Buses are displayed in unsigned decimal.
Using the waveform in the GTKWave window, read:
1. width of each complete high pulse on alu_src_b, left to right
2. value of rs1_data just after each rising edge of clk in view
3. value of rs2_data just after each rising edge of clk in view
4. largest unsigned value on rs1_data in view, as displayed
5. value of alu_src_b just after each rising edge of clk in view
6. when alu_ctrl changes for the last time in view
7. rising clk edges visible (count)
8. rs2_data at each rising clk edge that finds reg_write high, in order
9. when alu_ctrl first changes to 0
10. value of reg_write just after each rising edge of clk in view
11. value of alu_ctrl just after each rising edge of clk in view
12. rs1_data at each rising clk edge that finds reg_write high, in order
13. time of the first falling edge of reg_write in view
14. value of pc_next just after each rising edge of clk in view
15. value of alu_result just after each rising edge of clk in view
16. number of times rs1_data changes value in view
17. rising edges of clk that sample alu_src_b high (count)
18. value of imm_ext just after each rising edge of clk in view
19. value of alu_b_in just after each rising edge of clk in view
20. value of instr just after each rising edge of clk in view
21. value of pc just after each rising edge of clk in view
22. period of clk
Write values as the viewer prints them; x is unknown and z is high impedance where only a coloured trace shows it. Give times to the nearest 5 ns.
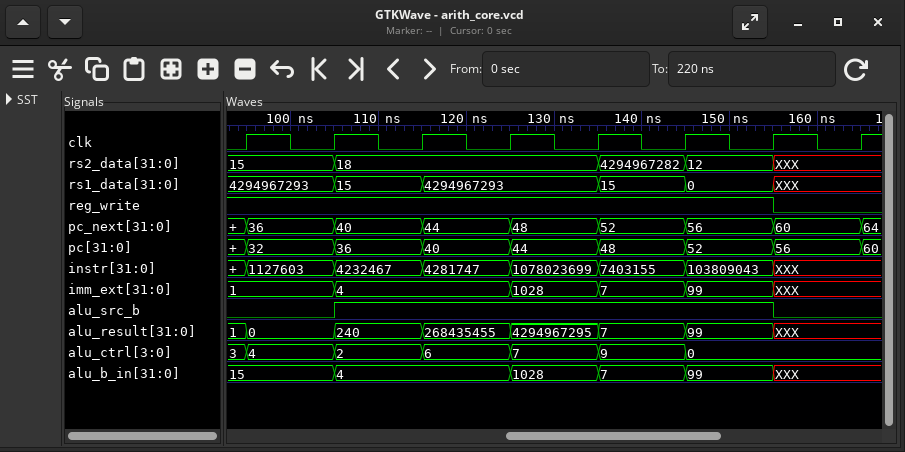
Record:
50 ns
4294967293, 15, 4294967293, 4294967293, 15, 0, XXX, XXX
15, 18, 18, 18, 4294967282, 12, XXX, XXX
4294967293
0 1 1 1 1 1 0 0
145 ns
8
15, 15, 18, 18, 18, 4294967282, 12
145 ns
1 1 1 1 1 1 0 0
4, 2, 6, 7, 9, 0, 0, 0
4294967293, 4294967293, 15, 4294967293, 4294967293, 15, 0
155 ns
36, 40, 44, 48, 52, 56, 60, 64
0, 240, 268435455, 4294967295, 7, 99, XXX, XXX
5
5
1, 4, 4, 1028, 7, 99, XXX, XXX
15, 4, 4, 1028, 7, 99, XXX, XXX
1127603, 4232467, 4281747, 1078023699, 7403155, 103809043, XXX, XXX
32, 36, 40, 44, 48, 52, 56, 60
10 ns
